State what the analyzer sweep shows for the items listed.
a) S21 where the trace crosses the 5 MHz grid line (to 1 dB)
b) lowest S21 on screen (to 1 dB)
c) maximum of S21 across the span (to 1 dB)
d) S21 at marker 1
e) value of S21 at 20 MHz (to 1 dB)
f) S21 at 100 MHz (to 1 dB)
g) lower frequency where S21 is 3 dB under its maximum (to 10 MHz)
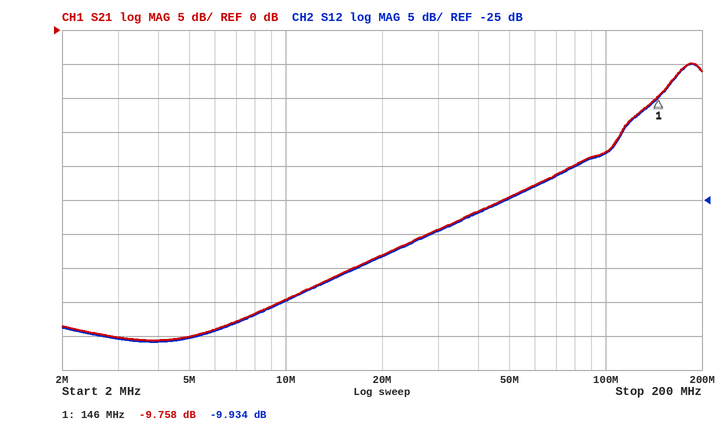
-45 dB
-46 dB
-5 dB
-9.758 dB
-33 dB
-18 dB
160 MHz
